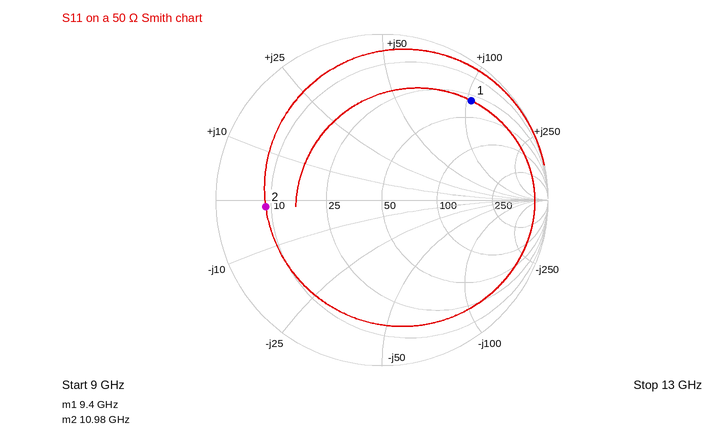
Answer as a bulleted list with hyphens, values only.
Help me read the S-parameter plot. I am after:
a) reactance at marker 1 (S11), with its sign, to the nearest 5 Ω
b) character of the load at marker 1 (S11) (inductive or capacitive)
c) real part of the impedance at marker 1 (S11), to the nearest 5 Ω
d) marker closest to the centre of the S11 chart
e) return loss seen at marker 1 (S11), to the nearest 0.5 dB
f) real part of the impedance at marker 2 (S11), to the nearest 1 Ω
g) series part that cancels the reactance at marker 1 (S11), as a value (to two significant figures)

- +105 Ω
- inductive
- 30 Ω
- marker 2
- 2.0 dB
- 9 Ω
- 160 fF
